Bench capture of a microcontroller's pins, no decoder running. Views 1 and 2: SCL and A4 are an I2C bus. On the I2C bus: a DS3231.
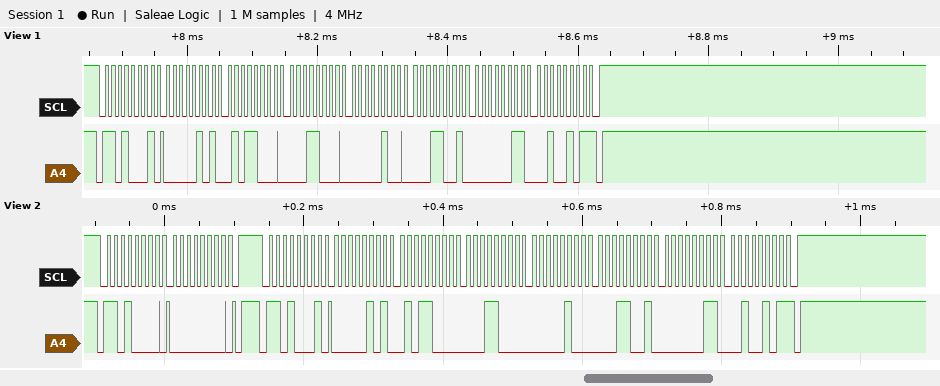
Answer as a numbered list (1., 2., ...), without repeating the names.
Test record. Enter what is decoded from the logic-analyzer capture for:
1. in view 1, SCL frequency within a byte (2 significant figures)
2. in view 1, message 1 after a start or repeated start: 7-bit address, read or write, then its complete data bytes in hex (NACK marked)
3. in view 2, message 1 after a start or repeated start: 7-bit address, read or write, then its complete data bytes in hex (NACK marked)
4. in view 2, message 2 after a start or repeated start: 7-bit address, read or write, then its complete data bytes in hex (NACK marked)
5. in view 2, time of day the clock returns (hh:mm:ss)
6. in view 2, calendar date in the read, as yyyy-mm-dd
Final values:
1. 100 kHz
2. 0x68 read: 05 58 18 04 19 03 25 NACK
3. 0x68 write: 00
4. 0x68 read: 05 58 18 04 19 03 25 NACK
5. 18:58:05
6. 2025-03-19
